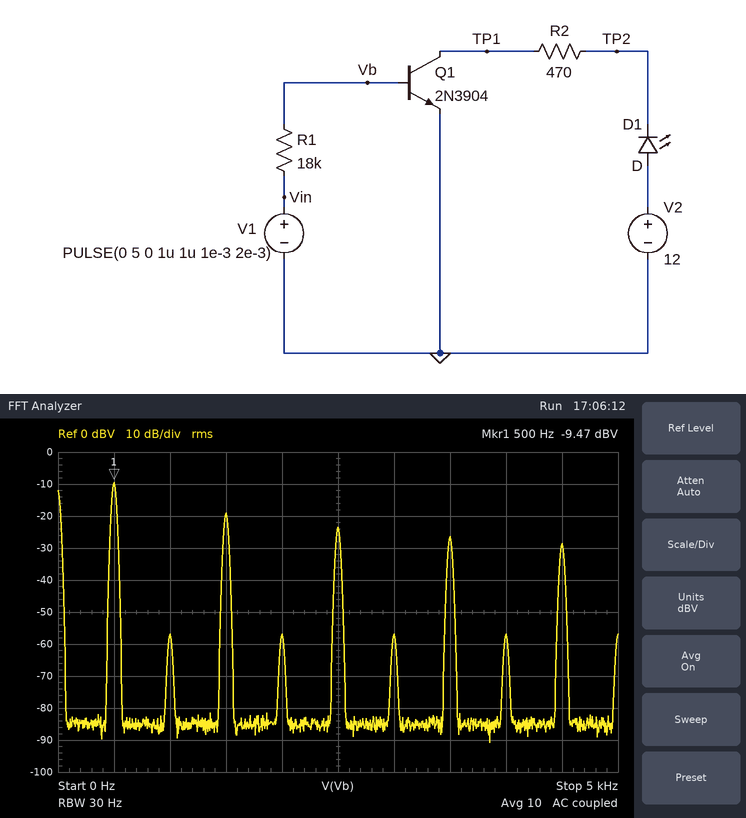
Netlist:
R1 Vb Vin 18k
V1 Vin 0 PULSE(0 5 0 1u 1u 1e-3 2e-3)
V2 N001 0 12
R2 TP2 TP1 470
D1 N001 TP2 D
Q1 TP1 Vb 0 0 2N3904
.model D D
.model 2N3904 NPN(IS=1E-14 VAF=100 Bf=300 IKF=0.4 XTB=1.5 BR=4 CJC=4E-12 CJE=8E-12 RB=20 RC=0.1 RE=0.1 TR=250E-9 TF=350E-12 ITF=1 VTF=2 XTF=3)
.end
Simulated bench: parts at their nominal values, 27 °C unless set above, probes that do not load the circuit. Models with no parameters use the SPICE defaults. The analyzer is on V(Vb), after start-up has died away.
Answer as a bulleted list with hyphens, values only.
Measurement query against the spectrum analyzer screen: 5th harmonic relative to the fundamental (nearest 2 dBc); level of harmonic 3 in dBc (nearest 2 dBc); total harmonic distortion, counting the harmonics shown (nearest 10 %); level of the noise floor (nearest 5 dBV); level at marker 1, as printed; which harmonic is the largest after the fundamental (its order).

- -14 dBc
- -10 dBc
- 40 %
- -85 dBV
- -9.47 dBV
- 3
